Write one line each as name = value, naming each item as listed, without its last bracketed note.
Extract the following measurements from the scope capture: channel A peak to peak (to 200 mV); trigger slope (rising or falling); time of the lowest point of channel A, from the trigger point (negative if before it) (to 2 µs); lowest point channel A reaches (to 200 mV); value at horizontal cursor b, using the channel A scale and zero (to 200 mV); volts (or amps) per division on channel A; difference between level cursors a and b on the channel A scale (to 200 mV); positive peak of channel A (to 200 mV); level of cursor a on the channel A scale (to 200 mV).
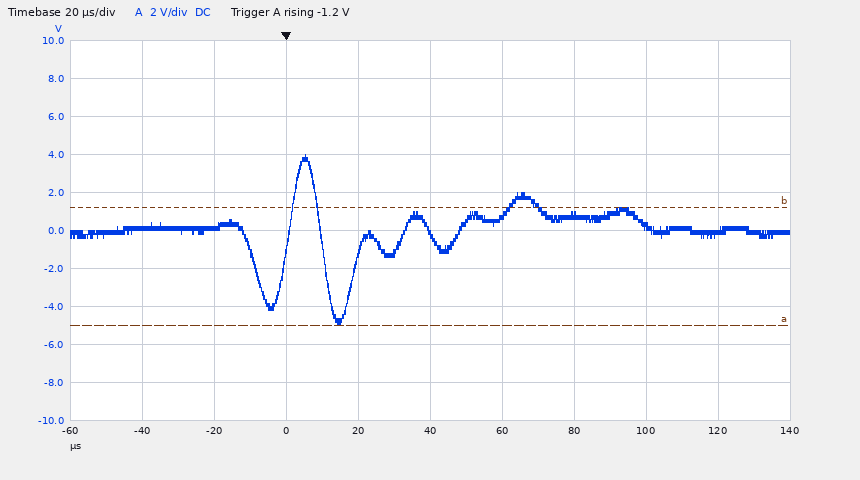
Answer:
channel A peak to peak = 9.0 V
trigger slope = rising
time of the lowest point of channel A, from the trigger point (negative if before it) = +14 µs
lowest point channel A reaches = -5.0 V
value at horizontal cursor b, using the channel A scale and zero = 1.2 V
volts (or amps) per division on channel A = 2 V
difference between level cursors a and b on the channel A scale = 6.2 V
positive peak of channel A = 4.0 V
level of cursor a on the channel A scale = -5.0 V
